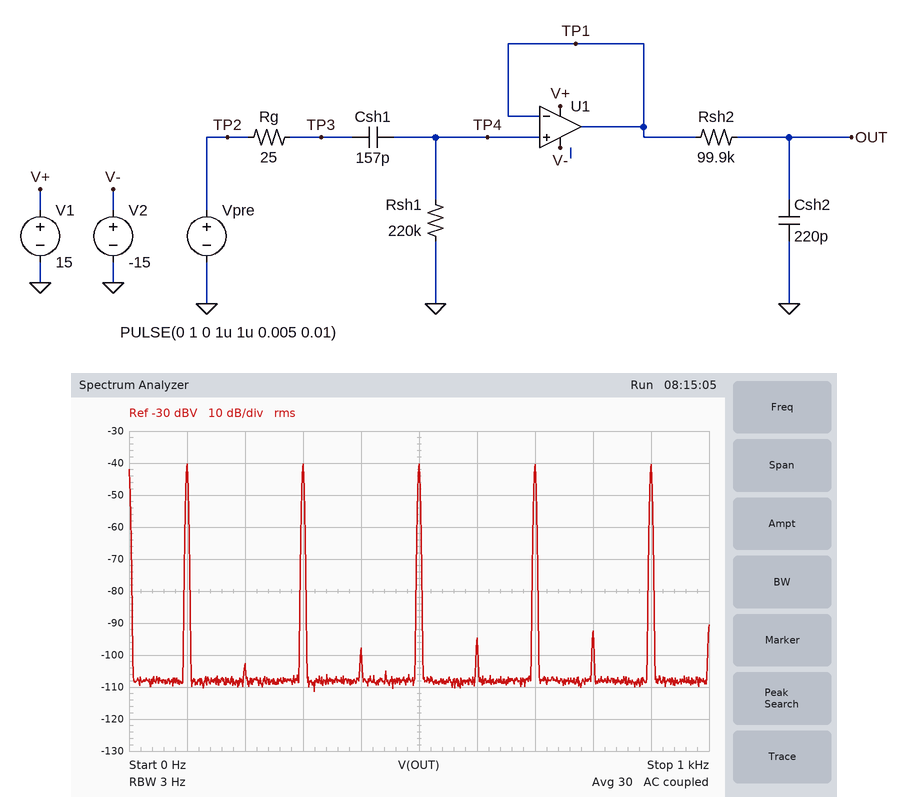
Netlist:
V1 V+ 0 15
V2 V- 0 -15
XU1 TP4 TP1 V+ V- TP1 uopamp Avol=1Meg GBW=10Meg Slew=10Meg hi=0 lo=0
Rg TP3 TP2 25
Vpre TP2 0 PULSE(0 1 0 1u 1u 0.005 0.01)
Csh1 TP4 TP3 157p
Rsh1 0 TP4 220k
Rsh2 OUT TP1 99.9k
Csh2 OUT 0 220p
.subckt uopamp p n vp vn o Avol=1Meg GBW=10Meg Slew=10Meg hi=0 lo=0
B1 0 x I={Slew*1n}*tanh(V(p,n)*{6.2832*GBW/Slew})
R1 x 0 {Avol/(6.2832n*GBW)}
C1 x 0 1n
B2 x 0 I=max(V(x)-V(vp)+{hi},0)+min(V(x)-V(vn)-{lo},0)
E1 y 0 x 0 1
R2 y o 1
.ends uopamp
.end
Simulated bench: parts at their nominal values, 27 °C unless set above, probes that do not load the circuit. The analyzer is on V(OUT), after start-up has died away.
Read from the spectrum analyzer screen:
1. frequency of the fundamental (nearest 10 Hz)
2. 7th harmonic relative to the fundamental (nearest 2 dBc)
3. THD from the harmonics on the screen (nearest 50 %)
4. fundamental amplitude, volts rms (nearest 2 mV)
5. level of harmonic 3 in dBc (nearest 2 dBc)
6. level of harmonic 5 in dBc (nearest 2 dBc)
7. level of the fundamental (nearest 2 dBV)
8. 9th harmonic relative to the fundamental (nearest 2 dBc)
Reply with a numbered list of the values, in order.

1. 100 Hz
2. 0 dBc
3. 200 %
4. 10 mV
5. 0 dBc
6. 0 dBc
7. -40 dBV
8. 0 dBc
